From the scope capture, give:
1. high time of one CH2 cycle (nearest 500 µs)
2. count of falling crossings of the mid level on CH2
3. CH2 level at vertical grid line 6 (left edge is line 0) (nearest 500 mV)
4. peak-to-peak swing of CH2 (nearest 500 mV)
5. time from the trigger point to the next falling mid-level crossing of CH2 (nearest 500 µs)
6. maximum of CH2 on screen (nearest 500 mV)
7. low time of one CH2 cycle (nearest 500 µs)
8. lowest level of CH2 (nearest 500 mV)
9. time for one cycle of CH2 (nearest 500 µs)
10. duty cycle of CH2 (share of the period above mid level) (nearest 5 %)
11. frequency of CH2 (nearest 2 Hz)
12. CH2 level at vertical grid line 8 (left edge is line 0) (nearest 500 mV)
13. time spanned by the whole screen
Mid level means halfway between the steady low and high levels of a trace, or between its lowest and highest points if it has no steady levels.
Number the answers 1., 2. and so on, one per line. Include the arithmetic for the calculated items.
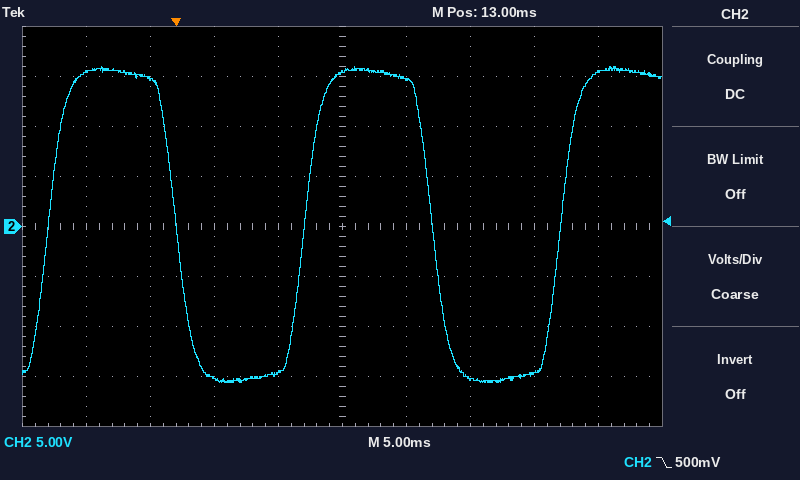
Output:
1. 10.0 ms
2. 2
3. 15.0 V
4. 16.0 V − (-15.5 V) = 31.5 V
5. 20.0 ms
6. 16.0 V
7. 10.0 ms
8. -15.5 V
9. 20.0 ms
10. 10.0 ms / 20.0 ms ≈ 50 %
11. 1 / 20.0 ms ≈ 50 Hz
12. -14.5 V
13. 50 ms
